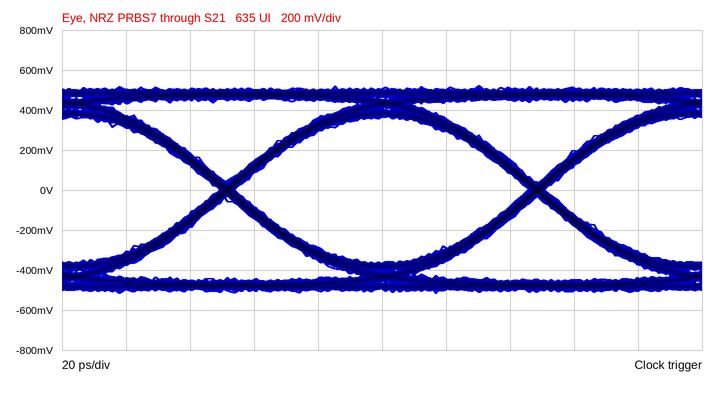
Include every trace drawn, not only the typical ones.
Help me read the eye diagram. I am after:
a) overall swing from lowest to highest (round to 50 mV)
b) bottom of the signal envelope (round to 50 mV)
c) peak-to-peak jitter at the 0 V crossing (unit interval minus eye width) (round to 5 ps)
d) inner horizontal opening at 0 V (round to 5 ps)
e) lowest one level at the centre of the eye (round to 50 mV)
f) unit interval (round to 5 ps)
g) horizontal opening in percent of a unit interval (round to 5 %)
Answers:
1.05 V
-500 mV
5 ps
90 ps
350 mV
95 ps
95 %
